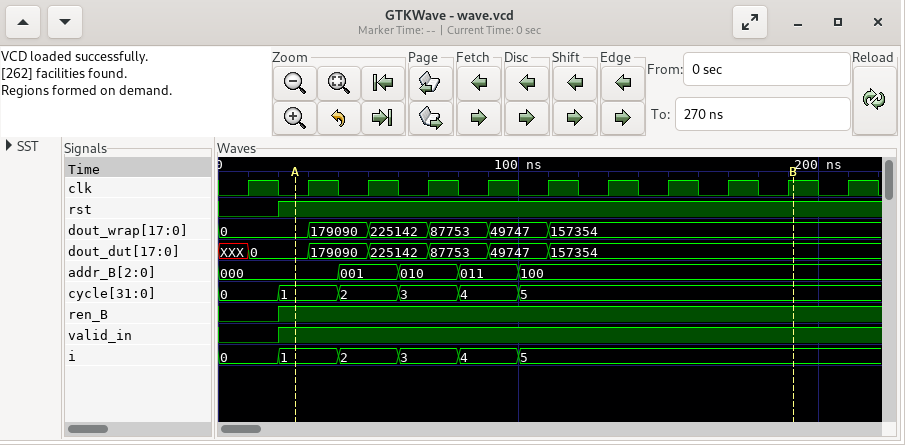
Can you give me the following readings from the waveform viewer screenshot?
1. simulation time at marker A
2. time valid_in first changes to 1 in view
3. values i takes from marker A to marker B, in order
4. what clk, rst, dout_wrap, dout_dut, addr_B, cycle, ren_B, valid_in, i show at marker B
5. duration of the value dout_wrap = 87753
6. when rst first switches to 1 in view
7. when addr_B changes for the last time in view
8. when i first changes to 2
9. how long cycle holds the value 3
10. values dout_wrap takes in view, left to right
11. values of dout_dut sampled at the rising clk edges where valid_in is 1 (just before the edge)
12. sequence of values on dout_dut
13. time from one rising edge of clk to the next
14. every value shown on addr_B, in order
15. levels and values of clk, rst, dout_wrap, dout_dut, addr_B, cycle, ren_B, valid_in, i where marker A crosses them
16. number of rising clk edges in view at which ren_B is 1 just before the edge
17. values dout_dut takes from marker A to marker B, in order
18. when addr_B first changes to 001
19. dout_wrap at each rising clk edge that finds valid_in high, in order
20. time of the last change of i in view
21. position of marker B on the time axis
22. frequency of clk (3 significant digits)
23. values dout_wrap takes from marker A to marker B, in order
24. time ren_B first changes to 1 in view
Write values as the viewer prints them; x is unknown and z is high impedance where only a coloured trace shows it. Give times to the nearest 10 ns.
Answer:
30 ns
20 ns
1, 2, 3, 4, 5
clk=1, rst=1, dout_wrap=157354, dout_dut=157354, addr_B=100, cycle=5, ren_B=1, valid_in=1, i=5
20 ns
20 ns
100 ns
40 ns
20 ns
0, 179090, 225142, 87753, 49747, 157354
0, 179090, 225142, 87753, 49747, 157354, 157354, 157354, 157354, 157354
XXX, 0, 179090, 225142, 87753, 49747, 157354
20 ns
000, 001, 010, 011, 100
clk=0, rst=1, dout_wrap=0, dout_dut=0, addr_B=000, cycle=1, ren_B=1, valid_in=1, i=1
10
0, 179090, 225142, 87753, 49747, 157354
40 ns
0, 179090, 225142, 87753, 49747, 157354, 157354, 157354, 157354, 157354
100 ns
190 ns
50.0 MHz
0, 179090, 225142, 87753, 49747, 157354
20 ns
